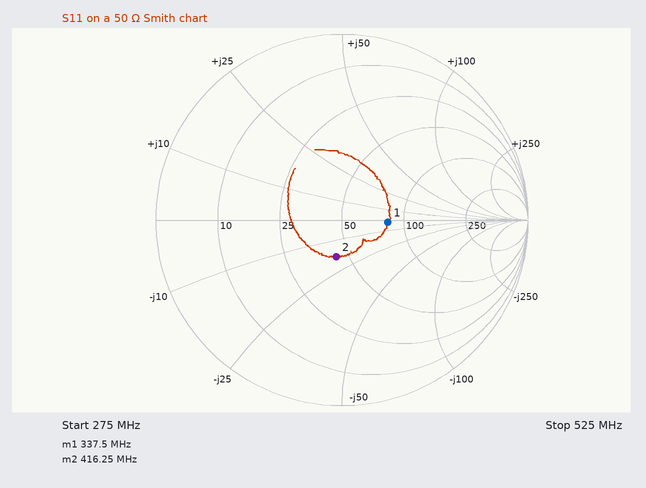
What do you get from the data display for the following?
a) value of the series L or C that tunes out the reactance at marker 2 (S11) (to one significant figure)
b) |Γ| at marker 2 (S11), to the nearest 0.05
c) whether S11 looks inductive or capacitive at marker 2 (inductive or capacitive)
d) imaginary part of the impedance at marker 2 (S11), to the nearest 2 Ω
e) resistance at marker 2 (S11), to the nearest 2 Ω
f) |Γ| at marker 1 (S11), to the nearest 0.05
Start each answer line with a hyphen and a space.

- 7 nH
- 0.20
- capacitive
- -18 Ω
- 44 Ω
- 0.25
